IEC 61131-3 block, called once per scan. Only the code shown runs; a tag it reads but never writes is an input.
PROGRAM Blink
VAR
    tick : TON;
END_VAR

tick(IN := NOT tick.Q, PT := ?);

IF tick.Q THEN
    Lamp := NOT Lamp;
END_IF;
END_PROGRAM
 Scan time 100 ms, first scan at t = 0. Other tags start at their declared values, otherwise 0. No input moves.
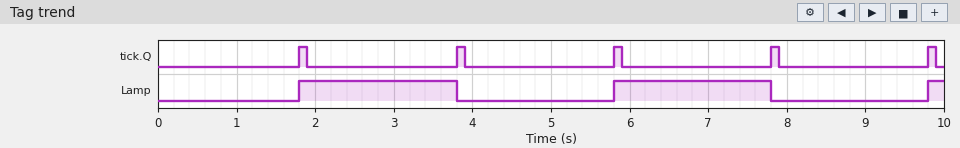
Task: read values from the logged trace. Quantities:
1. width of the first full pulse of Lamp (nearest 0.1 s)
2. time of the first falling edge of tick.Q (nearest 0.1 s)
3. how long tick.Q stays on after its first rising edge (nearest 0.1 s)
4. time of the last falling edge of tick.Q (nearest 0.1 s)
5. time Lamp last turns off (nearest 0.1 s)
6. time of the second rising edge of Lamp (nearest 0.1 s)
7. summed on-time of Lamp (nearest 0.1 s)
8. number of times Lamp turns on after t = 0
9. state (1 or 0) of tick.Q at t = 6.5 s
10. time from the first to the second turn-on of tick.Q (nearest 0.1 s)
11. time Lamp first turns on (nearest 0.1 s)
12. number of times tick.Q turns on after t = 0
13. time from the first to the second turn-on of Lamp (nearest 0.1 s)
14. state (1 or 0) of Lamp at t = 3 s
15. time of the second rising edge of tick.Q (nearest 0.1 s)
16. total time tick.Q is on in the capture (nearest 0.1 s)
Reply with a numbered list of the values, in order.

1. 2.0 s
2. 1.9 s
3. 0.1 s
4. 9.9 s
5. 7.8 s
6. 5.8 s
7. 4.2 s
8. 3
9. 0
10. 2.0 s
11. 1.8 s
12. 5
13. 4.0 s
14. 1
15. 3.8 s
16. 0.5 s
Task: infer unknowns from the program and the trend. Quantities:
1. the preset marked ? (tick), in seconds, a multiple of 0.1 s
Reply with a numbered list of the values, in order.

1. 1.8 s
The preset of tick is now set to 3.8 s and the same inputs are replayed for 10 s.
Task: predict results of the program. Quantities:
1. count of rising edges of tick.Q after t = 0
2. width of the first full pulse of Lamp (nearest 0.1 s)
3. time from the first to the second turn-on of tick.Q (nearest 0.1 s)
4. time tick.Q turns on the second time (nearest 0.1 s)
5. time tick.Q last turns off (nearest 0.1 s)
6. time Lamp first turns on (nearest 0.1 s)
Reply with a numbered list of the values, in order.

1. 2
2. 4.0 s
3. 4.0 s
4. 7.8 s
5. 7.9 s
6. 3.8 s
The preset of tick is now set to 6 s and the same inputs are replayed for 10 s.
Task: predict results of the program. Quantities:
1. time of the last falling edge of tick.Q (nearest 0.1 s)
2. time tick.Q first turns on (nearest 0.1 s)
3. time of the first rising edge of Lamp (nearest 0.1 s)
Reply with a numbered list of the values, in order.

1. 6.1 s
2. 6.0 s
3. 6.0 s
